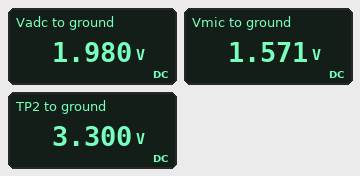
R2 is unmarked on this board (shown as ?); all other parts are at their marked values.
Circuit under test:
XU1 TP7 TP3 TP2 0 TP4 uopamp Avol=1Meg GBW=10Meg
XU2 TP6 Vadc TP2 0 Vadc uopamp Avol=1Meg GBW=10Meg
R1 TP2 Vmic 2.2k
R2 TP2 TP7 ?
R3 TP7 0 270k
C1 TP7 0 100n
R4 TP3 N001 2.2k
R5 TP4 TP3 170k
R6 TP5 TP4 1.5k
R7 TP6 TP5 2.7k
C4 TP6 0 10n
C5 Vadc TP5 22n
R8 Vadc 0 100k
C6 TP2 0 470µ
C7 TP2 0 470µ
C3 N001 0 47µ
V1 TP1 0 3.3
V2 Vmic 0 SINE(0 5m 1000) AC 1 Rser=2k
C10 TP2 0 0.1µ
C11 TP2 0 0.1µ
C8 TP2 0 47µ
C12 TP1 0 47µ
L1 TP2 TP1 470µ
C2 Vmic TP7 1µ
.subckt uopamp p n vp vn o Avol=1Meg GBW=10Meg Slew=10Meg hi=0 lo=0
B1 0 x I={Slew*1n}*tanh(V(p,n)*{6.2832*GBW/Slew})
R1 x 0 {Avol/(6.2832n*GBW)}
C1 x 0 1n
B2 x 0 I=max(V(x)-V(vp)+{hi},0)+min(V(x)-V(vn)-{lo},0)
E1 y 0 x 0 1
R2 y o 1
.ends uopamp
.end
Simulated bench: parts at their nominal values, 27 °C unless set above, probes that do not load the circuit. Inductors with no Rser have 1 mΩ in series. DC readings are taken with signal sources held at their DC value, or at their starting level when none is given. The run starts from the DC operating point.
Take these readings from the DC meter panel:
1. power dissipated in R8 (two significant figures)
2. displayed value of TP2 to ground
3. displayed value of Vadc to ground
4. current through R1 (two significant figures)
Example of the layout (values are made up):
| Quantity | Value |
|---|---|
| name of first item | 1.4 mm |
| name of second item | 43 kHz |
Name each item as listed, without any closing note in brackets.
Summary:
| Quantity | Value |
|---|---|
| power dissipated in R8 | 39 µW |
| displayed value of TP2 to ground | 3.300 V |
| displayed value of Vadc to ground | 1.980 V |
| current through R1 | 790 µA |
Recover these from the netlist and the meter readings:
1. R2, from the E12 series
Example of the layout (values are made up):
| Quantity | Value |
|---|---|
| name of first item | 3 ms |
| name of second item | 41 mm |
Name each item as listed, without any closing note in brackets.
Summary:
| Quantity | Value |
|---|---|
| R2, from the E12 series | 180 kΩ |
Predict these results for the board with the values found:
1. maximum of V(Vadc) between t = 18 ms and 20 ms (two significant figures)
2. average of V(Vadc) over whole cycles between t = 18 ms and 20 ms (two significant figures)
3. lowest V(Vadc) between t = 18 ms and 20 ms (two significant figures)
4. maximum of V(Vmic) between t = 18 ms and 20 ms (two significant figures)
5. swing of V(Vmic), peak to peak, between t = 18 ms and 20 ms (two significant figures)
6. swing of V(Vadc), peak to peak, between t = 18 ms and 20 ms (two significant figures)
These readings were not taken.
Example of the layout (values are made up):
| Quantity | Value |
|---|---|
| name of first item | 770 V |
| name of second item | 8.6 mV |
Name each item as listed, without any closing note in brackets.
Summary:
| Quantity | Value |
|---|---|
| maximum of V(Vadc) between t = 18 ms and 20 ms | 2.1 V |
| average of V(Vadc) over whole cycles between t = 18 ms and 20 ms | 2.0 V |
| lowest V(Vadc) between t = 18 ms and 20 ms | 1.8 V |
| maximum of V(Vmic) between t = 18 ms and 20 ms | 1.6 V |
| swing of V(Vmic), peak to peak, between t = 18 ms and 20 ms | 4.5 mV |
| swing of V(Vadc), peak to peak, between t = 18 ms and 20 ms | 320 mV |
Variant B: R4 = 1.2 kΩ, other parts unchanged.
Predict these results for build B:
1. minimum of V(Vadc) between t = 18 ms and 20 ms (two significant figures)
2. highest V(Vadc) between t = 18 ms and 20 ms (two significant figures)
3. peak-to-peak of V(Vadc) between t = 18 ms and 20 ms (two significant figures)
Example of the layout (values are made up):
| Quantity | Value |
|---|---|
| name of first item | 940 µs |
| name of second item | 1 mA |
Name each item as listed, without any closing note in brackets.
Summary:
| Quantity | Value |
|---|---|
| minimum of V(Vadc) between t = 18 ms and 20 ms | 1.7 V |
| highest V(Vadc) between t = 18 ms and 20 ms | 2.3 V |
| peak-to-peak of V(Vadc) between t = 18 ms and 20 ms | 580 mV |
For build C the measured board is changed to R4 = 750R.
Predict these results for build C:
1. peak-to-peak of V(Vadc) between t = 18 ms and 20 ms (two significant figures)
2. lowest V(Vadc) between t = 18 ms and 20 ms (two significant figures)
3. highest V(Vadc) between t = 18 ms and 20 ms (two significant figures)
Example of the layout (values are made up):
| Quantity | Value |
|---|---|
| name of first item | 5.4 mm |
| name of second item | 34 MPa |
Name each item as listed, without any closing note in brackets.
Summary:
| Quantity | Value |
|---|---|
| peak-to-peak of V(Vadc) between t = 18 ms and 20 ms | 920 mV |
| lowest V(Vadc) between t = 18 ms and 20 ms | 1.5 V |
| highest V(Vadc) between t = 18 ms and 20 ms | 2.4 V |
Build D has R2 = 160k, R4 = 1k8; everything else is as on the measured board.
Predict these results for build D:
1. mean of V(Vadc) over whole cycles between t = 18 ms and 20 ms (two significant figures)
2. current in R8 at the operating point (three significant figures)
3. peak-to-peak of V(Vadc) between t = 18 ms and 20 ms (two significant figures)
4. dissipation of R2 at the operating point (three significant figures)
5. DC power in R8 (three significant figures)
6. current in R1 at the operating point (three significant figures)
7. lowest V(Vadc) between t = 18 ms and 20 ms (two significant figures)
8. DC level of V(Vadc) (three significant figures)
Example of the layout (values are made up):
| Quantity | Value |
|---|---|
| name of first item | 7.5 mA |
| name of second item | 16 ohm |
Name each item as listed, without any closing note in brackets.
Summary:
| Quantity | Value |
|---|---|
| mean of V(Vadc) over whole cycles between t = 18 ms and 20 ms | 2.1 V |
| current in R8 at the operating point | 20.7 µA |
| peak-to-peak of V(Vadc) between t = 18 ms and 20 ms | 390 mV |
| dissipation of R2 at the operating point | 9.42 µW |
| DC power in R8 | 42.9 µW |
| current in R1 at the operating point | 786 µA |
| lowest V(Vadc) between t = 18 ms and 20 ms | 1.9 V |
| DC level of V(Vadc) | 2.07 V |
